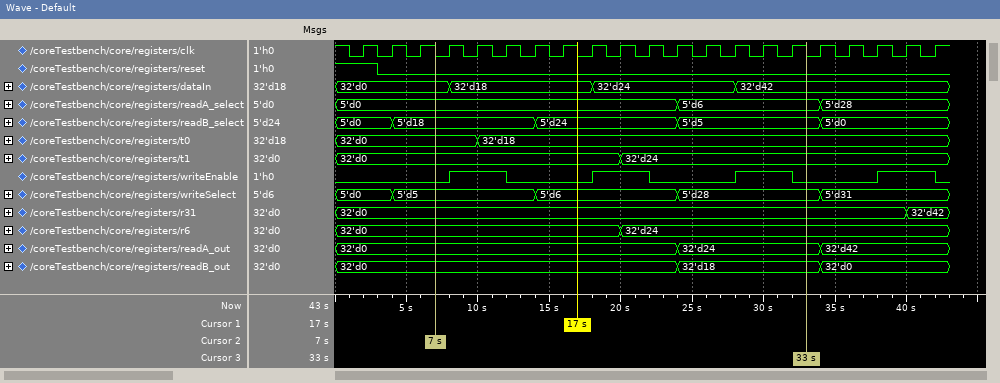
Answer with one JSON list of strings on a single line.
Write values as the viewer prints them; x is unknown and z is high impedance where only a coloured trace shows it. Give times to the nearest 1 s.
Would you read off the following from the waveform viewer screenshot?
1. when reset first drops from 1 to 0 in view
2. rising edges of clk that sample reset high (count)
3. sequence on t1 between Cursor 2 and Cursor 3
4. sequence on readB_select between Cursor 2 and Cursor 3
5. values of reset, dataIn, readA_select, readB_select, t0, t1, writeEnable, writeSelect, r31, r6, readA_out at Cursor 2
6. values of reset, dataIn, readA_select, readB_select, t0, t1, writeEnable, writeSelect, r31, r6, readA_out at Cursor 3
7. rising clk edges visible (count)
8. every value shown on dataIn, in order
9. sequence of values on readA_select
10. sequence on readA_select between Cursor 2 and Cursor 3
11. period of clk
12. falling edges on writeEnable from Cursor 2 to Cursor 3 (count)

["3 s", "1", "32'd0, 32'd24", "5'd18, 5'd24, 5'd5", "reset=0, dataIn=32'd0, readA_select=5'd0, readB_select=5'd18, t0=32'd0, t1=32'd0, writeEnable=0, writeSelect=5'd5, r31=32'd0, r6=32'd0, readA_out=32'd0", "reset=0, dataIn=32'd42, readA_select=5'd6, readB_select=5'd5, t0=32'd18, t1=32'd24, writeEnable=0, writeSelect=5'd28, r31=32'd0, r6=32'd24, readA_out=32'd24", "21", "32'd0, 32'd18, 32'd24, 32'd42", "5'd0, 5'd6, 5'd28", "5'd0, 5'd6", "2 s", "3"]
